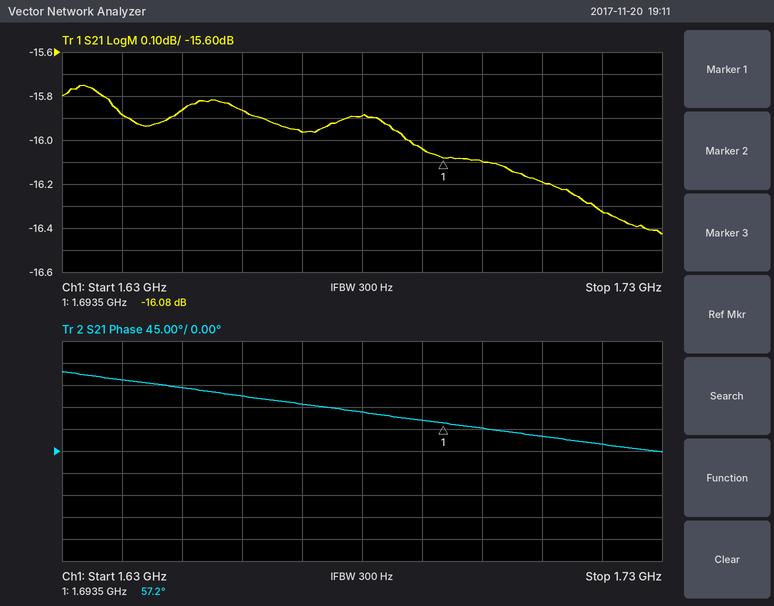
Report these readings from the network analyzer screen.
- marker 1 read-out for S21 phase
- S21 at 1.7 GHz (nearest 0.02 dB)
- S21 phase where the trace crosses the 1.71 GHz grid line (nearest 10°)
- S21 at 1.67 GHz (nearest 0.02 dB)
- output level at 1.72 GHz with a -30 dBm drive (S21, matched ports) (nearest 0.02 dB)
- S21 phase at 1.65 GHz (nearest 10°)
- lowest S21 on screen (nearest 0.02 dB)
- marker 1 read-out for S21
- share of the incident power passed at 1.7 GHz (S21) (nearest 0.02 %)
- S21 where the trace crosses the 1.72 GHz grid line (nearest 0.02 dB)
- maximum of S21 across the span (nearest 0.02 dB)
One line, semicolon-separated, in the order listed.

57.2°; -16.10 dB; 30°; -15.96 dB; -46.32 dBm; 130°; -16.42 dB; -16.08 dB; 2.46 %; -16.32 dB; -15.76 dB
